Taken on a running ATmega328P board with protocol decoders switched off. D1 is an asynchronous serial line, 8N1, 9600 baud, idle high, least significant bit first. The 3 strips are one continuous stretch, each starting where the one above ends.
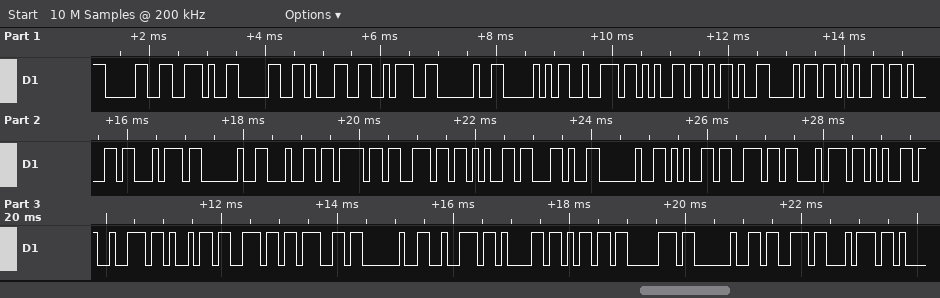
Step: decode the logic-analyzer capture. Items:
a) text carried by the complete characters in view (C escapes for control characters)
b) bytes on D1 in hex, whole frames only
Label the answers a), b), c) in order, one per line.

a) "0.01: Pre-heat done, entering ramp st"
b) 0x30 0x2E 0x30 0x31 0x3A 0x20 0x50 0x72 0x65 0x2D 0x68 0x65 0x61 0x74 0x20 0x64 0x6F 0x6E 0x65 0x2C 0x20 0x65 0x6E 0x74 0x65 0x72 0x69 0x6E 0x67 0x20 0x72 0x61 0x6D 0x70 0x20 0x73 0x74
